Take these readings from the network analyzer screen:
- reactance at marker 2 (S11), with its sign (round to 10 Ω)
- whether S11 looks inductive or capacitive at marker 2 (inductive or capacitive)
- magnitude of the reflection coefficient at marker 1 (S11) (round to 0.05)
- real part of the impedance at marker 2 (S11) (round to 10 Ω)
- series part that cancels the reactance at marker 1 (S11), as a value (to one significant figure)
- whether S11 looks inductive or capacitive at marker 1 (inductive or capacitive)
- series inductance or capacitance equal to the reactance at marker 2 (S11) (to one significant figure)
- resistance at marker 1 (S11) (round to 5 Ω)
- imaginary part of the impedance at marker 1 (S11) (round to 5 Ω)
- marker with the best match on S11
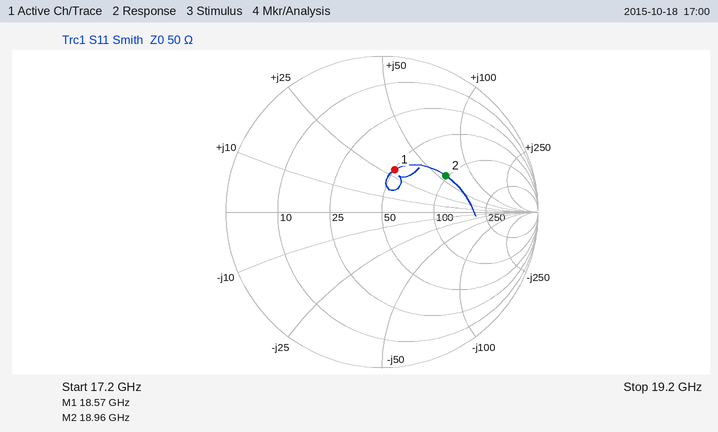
+60 Ω
inductive
0.30
100 Ω
300 fF
inductive
500 pH
50 Ω
+30 Ω
marker 1
